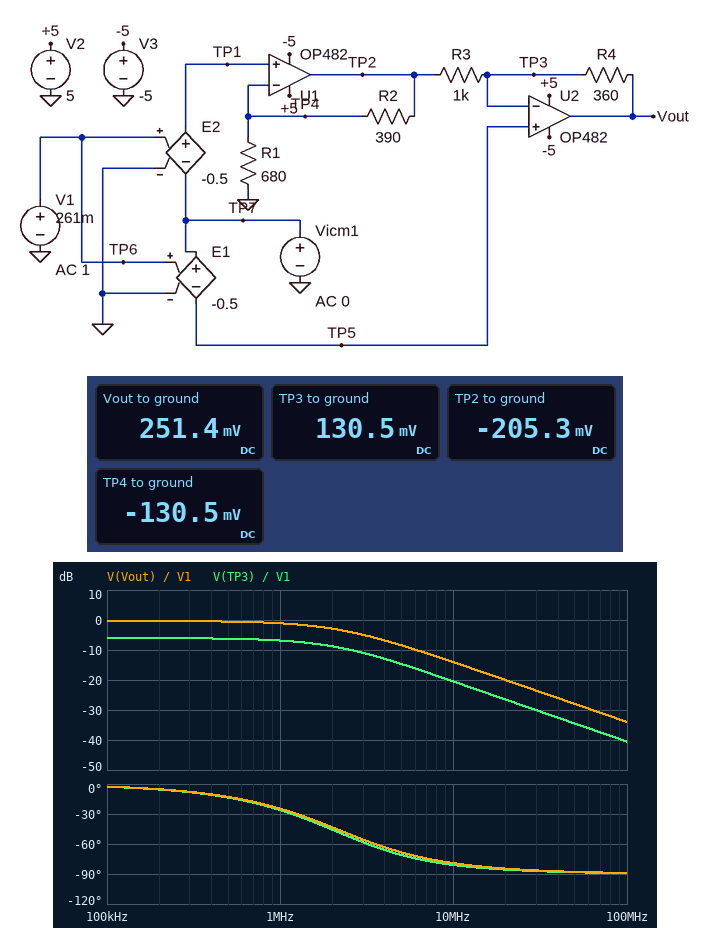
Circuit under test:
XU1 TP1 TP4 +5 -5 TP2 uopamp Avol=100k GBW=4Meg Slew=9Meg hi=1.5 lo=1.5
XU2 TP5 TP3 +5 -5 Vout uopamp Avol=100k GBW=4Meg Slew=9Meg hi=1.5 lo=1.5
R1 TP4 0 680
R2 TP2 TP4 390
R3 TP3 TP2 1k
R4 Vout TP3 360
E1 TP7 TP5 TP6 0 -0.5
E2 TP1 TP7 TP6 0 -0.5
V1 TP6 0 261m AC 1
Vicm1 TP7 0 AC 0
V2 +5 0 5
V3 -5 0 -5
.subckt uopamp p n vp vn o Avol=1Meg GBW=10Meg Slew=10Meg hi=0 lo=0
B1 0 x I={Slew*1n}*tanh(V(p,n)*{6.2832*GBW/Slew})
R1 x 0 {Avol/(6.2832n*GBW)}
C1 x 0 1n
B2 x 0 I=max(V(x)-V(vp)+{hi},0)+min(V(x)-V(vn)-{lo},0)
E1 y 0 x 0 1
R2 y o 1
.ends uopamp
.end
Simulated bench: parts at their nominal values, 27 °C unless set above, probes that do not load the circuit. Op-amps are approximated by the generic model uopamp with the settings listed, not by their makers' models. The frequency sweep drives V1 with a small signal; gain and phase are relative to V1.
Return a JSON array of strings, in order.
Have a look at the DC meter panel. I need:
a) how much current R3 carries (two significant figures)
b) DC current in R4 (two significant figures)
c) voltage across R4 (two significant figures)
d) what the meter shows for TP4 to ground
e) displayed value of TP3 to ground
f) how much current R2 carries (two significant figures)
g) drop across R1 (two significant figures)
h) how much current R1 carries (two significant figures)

["340 µA", "340 µA", "120 mV", "-130.5 mV", "130.5 mV", "190 µA", "130 mV", "190 µA"]
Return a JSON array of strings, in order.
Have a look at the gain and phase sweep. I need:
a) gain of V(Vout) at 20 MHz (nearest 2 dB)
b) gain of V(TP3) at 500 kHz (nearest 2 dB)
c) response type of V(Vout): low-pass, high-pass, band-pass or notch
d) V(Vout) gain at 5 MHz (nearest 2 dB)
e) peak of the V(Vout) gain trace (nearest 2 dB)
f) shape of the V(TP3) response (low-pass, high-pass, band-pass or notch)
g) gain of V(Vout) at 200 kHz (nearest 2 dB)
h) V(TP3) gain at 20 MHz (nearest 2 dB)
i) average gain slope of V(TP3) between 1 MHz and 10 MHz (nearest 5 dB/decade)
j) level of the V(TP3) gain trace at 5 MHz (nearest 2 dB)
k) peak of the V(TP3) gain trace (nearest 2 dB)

["-20 dB", "-6 dB", "low-pass", "-8 dB", "0 dB", "low-pass", "0 dB", "-26 dB", "-15 dB/decade", "-14 dB", "-6 dB"]
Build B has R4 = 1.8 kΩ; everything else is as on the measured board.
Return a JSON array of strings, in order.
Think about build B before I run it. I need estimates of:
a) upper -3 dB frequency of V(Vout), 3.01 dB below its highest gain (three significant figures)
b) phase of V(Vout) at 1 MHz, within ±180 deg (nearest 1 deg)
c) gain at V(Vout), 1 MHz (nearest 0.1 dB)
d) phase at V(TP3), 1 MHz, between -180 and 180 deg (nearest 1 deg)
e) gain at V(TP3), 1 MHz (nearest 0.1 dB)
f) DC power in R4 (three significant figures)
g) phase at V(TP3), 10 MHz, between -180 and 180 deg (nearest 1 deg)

["1.21 MHz", "-45 deg", "6.8 dB", "-74 deg", "-8.0 dB", "203 µW", "130 deg"]
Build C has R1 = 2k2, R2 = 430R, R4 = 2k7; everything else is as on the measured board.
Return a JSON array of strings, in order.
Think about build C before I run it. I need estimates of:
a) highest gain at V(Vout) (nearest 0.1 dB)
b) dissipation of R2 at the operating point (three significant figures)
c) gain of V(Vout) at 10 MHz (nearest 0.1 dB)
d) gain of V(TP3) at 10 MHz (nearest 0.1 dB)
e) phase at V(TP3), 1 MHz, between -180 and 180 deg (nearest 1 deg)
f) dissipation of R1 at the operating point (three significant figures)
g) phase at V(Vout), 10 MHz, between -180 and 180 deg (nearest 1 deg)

["10.8 dB", "1.51 µW", "-13.1 dB", "-21.1 dB", "-86 deg", "7.74 µW", "-97 deg"]
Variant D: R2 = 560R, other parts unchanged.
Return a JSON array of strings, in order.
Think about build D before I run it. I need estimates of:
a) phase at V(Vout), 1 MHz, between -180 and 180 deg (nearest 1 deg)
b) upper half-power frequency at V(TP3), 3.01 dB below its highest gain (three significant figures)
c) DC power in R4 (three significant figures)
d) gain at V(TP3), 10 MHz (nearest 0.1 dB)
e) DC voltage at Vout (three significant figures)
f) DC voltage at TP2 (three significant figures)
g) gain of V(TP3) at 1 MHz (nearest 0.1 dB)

["-26 deg", "2.00 MHz", "48.9 µW", "-20.6 dB", "263 mV", "-238 mV", "-7.0 dB"]
